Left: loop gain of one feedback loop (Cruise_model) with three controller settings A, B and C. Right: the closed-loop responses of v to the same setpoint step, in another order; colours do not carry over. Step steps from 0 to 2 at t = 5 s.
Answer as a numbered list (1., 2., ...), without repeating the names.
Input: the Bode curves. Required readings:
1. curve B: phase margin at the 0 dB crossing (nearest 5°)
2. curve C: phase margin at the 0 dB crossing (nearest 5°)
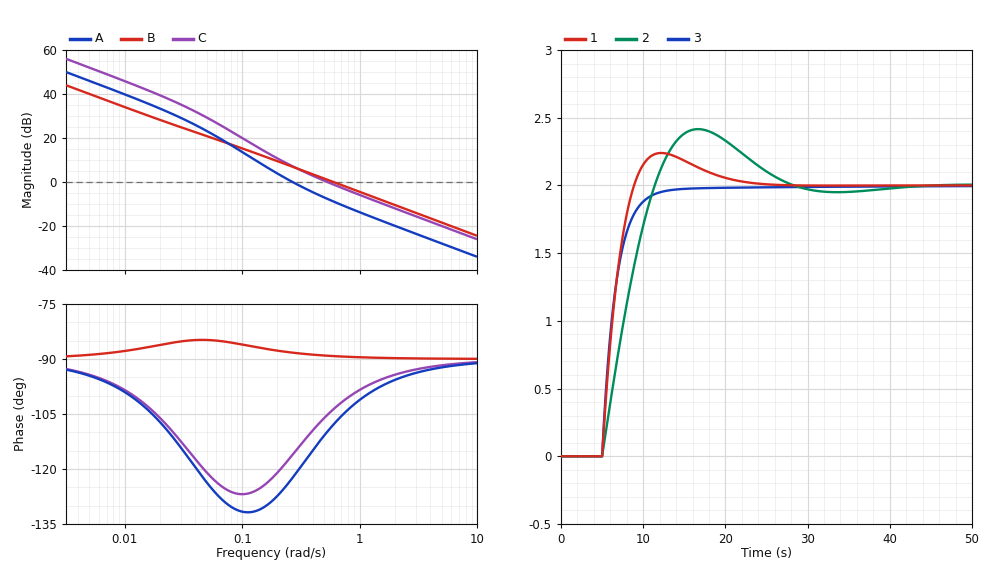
1. 90°
2. 75°
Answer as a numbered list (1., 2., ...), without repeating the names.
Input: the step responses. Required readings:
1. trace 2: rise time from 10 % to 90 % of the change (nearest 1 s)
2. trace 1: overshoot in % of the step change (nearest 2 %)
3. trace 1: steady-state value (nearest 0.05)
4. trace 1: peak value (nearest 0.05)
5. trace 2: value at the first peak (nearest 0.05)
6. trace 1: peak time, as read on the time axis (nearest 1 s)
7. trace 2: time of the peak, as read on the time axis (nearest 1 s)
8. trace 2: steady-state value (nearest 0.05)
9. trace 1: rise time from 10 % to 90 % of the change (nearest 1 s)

1. 5 s
2. 12 %
3. 2.00
4. 2.25
5. 2.40
6. 12 s
7. 17 s
8. 2.00
9. 3 s
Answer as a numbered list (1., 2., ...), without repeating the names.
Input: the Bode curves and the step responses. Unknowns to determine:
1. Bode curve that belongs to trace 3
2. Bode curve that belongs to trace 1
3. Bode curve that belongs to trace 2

1. B
2. C
3. A
